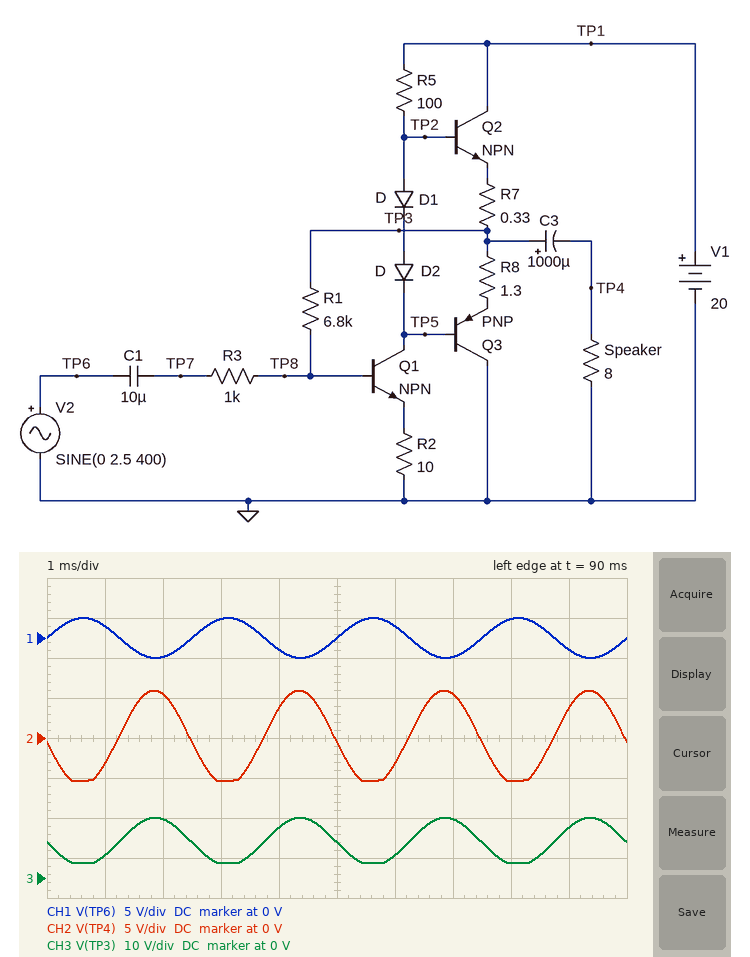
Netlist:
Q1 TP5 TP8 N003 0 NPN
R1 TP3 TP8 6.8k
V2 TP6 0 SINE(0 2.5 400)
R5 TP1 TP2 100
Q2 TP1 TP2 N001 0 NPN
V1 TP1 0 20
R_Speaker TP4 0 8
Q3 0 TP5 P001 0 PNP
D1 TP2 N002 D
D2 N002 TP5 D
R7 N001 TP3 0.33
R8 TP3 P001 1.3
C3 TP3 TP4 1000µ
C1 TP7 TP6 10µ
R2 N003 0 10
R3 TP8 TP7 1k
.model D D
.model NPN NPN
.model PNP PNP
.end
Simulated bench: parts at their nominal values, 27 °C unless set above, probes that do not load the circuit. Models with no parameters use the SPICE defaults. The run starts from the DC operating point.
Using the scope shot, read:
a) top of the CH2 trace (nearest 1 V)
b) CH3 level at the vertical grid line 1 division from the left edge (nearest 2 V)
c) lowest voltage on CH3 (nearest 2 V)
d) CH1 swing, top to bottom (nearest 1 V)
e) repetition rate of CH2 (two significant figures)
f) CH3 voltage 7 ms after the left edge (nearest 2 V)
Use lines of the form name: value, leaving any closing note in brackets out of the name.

top of the CH2 trace: 6 V
CH3 level at the vertical grid line 1 division from the left edge: 6 V
lowest voltage on CH3: 4 V
CH1 swing, top to bottom: 5 V
repetition rate of CH2: 400 Hz
CH3 voltage 7 ms after the left edge: 14 V
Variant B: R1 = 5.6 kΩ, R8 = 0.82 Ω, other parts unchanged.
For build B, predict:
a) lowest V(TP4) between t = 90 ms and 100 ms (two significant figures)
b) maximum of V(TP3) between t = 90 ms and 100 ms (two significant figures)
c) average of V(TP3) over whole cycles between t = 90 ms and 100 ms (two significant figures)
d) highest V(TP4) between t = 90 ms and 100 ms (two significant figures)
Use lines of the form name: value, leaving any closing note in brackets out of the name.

lowest V(TP4) between t = 90 ms and 100 ms: -5.0 V
maximum of V(TP3) between t = 90 ms and 100 ms: 14 V
average of V(TP3) over whole cycles between t = 90 ms and 100 ms: 8.3 V
highest V(TP4) between t = 90 ms and 100 ms: 5.5 V
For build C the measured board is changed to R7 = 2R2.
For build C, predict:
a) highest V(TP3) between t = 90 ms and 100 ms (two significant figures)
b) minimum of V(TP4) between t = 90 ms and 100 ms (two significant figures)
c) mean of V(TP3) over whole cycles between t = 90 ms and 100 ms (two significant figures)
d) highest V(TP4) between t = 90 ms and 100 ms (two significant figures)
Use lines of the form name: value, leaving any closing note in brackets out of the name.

highest V(TP3) between t = 90 ms and 100 ms: 14 V
minimum of V(TP4) between t = 90 ms and 100 ms: -5.3 V
mean of V(TP3) over whole cycles between t = 90 ms and 100 ms: 8.9 V
highest V(TP4) between t = 90 ms and 100 ms: 5.5 V
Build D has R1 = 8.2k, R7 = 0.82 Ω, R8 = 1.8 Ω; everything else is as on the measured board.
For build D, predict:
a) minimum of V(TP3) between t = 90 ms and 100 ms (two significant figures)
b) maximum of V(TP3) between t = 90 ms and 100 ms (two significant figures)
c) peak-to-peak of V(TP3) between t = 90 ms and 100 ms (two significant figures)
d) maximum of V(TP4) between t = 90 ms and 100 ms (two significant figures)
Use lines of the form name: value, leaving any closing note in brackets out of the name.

minimum of V(TP3) between t = 90 ms and 100 ms: 4.1 V
maximum of V(TP3) between t = 90 ms and 100 ms: 16 V
peak-to-peak of V(TP3) between t = 90 ms and 100 ms: 12 V
maximum of V(TP4) between t = 90 ms and 100 ms: 6.1 V
